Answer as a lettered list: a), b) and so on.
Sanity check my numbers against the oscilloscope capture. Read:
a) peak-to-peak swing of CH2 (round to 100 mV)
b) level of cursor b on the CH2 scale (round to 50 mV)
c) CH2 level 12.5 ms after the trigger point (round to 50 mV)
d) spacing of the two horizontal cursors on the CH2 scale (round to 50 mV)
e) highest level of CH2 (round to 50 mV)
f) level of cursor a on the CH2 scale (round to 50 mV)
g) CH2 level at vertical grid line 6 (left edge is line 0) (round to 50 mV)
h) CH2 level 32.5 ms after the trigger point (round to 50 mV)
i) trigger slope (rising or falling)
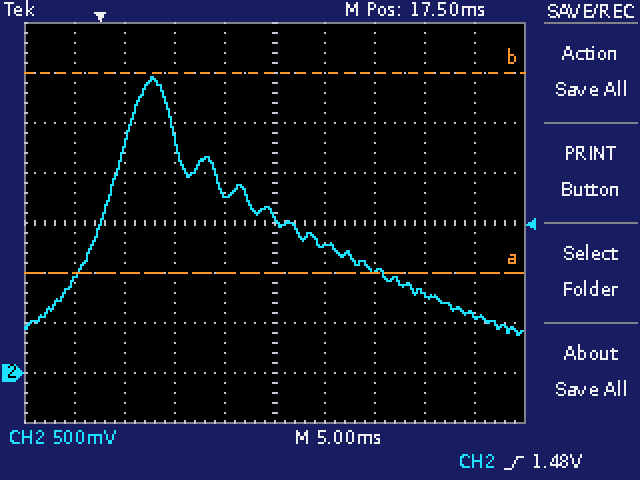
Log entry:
a) 2.60 V
b) 3.00 V
c) 1.80 V
d) 2.00 V
e) 2.95 V
f) 1.00 V
g) 1.25 V
h) 800 mV
i) rising
